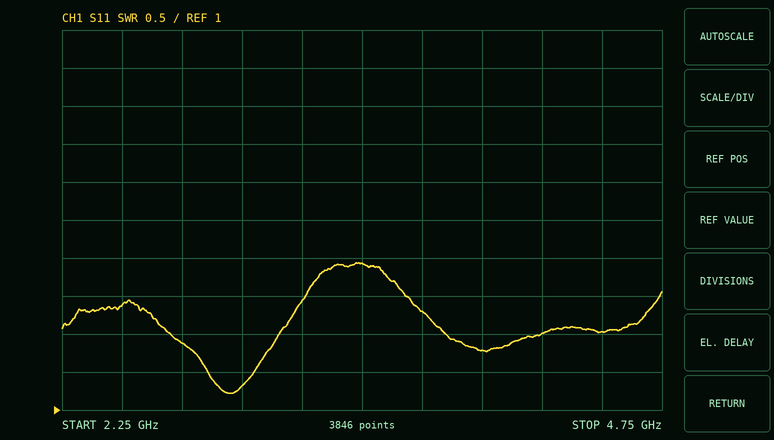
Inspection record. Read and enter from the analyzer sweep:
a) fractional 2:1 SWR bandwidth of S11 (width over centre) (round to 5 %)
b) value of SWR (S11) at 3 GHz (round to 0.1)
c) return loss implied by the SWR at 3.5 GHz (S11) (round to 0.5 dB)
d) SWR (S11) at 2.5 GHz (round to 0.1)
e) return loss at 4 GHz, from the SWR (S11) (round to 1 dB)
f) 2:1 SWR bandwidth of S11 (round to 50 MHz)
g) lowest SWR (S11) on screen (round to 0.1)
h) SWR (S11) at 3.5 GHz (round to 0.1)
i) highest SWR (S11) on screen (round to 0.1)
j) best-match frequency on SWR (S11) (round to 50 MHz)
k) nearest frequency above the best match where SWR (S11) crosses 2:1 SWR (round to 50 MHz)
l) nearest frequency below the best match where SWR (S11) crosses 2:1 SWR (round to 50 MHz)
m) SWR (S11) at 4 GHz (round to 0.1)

15 %
1.3
6.0 dB
2.4
11 dB
450 MHz
1.2
2.9
2.9
2.95 GHz
3.15 GHz
2.70 GHz
1.8
